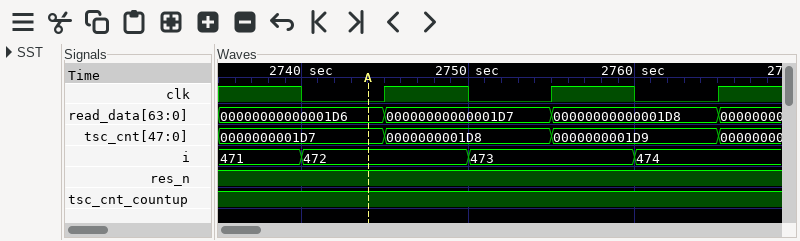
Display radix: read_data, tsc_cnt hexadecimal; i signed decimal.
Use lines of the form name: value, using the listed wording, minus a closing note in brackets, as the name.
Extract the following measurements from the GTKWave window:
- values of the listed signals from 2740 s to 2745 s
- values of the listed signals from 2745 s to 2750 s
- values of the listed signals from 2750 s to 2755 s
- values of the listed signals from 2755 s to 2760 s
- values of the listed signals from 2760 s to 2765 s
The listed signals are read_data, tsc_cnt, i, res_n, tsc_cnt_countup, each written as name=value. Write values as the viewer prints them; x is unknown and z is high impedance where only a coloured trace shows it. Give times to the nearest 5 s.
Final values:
values of the listed signals from 2740 s to 2745 s: read_data=00000000000001D6, tsc_cnt=0000000001D7, i=472, res_n=1, tsc_cnt_countup=1
values of the listed signals from 2745 s to 2750 s: read_data=00000000000001D7, tsc_cnt=0000000001D8, i=472, res_n=1, tsc_cnt_countup=1
values of the listed signals from 2750 s to 2755 s: read_data=00000000000001D7, tsc_cnt=0000000001D8, i=473, res_n=1, tsc_cnt_countup=1
values of the listed signals from 2755 s to 2760 s: read_data=00000000000001D8, tsc_cnt=0000000001D9, i=473, res_n=1, tsc_cnt_countup=1
values of the listed signals from 2760 s to 2765 s: read_data=00000000000001D8, tsc_cnt=0000000001D9, i=474, res_n=1, tsc_cnt_countup=1
